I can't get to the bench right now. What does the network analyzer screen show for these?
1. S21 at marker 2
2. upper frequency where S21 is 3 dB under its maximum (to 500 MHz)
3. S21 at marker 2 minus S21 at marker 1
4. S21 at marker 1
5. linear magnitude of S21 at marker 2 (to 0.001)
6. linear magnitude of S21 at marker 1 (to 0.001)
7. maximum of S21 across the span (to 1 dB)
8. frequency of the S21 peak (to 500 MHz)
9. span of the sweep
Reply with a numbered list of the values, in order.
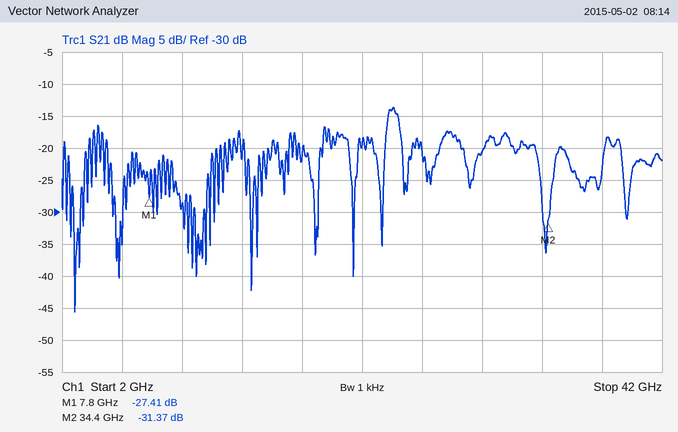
1. -31.37 dB
2. 24.5 GHz
3. -3.96 dB
4. -27.41 dB
5. 0.027
6. 0.043
7. -14 dB
8. 24.0 GHz
9. 40 GHz
